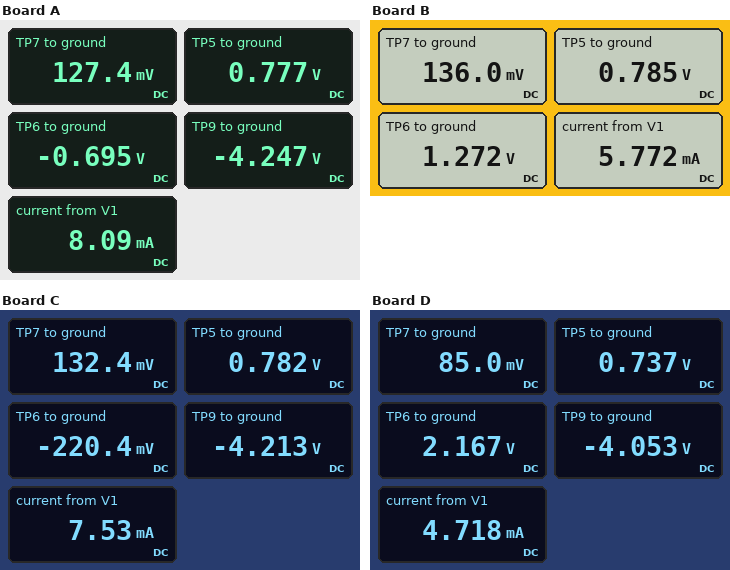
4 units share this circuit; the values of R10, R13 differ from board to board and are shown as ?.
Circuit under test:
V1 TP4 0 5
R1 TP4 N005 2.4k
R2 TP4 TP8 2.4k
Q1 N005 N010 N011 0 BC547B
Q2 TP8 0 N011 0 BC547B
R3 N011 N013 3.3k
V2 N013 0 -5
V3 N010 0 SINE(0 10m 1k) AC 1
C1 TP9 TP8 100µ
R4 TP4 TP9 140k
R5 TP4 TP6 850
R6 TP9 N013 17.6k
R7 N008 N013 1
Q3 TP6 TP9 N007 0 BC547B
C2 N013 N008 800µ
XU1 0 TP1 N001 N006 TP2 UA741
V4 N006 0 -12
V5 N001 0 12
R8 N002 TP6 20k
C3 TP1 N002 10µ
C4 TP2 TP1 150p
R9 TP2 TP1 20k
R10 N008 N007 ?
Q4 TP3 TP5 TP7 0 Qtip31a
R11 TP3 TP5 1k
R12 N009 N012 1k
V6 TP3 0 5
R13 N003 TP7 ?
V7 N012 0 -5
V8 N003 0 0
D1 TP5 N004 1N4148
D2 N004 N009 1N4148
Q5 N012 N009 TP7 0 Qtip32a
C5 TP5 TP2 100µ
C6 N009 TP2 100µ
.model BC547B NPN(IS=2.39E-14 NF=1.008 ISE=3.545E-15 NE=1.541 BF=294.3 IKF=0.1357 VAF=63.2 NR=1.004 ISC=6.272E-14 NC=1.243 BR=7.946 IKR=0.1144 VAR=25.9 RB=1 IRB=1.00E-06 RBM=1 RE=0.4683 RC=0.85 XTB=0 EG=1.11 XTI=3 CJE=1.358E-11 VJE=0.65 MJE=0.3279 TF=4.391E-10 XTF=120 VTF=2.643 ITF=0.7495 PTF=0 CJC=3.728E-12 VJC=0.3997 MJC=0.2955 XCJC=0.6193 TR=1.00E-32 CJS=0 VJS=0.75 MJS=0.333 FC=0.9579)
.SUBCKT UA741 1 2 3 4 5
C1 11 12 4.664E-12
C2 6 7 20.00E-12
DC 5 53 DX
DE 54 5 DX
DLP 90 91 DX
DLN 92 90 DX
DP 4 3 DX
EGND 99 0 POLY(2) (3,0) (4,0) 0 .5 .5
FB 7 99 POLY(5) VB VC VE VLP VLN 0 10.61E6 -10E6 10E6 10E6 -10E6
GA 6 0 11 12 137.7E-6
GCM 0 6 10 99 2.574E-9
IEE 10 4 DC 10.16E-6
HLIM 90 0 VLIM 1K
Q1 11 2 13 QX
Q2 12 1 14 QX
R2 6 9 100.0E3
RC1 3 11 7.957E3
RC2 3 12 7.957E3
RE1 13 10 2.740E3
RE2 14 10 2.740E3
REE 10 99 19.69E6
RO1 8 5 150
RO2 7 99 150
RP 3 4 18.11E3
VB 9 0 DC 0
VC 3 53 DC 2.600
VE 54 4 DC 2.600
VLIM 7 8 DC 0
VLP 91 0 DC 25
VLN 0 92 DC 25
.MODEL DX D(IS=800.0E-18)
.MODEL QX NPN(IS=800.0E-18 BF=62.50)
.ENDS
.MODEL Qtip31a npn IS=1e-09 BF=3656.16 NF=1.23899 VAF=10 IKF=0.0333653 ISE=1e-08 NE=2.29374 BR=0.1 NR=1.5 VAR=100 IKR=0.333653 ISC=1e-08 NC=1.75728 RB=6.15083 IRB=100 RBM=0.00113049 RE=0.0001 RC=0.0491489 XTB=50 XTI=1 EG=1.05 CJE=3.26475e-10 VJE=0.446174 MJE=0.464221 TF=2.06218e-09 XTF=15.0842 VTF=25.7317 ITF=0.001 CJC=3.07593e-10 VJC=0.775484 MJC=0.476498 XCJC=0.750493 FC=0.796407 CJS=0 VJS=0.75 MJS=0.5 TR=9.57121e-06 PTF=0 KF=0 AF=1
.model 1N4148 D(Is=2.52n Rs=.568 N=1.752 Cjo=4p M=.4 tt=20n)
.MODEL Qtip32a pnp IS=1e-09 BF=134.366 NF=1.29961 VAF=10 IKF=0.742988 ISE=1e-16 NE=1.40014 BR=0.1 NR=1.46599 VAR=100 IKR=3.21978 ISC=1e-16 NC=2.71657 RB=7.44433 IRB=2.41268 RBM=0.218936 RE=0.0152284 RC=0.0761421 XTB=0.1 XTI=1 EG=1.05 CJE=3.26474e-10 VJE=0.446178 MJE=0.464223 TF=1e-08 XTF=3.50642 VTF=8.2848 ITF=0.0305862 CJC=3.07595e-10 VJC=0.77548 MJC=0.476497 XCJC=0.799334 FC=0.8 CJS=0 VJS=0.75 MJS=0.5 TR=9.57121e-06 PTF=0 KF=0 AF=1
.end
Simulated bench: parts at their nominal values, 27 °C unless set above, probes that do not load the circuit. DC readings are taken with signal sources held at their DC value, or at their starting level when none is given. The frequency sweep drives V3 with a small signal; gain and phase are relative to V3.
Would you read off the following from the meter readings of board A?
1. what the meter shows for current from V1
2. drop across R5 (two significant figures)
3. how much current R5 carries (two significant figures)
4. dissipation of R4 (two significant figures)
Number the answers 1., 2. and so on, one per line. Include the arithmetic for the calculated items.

1. 8.09 mA
2. 5 V - (-695 mV) = 5.7 V
3. (5 V - (-695 mV)) / 850 Ω = 6.7 mA
4. (5 V - (-4.247 V))^2 / 140 kΩ = 610 µW
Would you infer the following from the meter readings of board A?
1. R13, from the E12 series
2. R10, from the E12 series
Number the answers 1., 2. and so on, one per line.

1. 12 Ω
2. 8.2 Ω
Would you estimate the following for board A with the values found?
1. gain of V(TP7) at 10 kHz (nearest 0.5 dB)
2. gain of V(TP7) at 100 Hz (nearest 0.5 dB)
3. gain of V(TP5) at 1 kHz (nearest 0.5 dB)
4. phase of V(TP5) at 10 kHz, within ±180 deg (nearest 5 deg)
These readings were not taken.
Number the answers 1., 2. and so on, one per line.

1. 59.5 dB
2. 59.0 dB
3. 59.5 dB
4. -15 deg
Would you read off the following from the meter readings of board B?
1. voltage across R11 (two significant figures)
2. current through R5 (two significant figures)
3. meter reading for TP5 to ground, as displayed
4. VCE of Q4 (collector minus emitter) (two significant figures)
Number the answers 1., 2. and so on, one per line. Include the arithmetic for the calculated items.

1. 5 V - 785 mV = 4.2 V
2. (5 V - 1.272 V) / 850 Ω = 4.4 mA
3. 0.785 V
4. 5 V - 136 mV = 4.9 V
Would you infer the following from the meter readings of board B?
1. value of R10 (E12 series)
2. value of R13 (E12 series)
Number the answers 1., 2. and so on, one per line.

1. 47 Ω
2. 18 Ω
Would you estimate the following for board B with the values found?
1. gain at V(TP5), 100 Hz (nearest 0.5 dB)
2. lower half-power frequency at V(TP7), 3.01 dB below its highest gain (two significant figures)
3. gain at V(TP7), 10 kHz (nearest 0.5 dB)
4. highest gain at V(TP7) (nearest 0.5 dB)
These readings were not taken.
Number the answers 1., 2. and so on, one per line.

1. 50.5 dB
2. 2.3 Hz
3. 50.0 dB
4. 50.5 dB
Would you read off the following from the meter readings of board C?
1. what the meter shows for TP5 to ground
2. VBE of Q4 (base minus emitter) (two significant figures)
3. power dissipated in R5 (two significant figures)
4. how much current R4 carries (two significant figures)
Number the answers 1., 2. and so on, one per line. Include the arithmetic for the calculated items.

1. 0.782 V
2. 782 mV - 132.4 mV = 650 mV
3. (5 V - (-220.4 mV))^2 / 850 Ω = 32 mW
4. (5 V - (-4.213 V)) / 140 kΩ = 66 µA
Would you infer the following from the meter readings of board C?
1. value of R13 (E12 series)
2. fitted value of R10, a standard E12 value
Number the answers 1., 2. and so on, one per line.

1. 15 Ω
2. 15 Ω
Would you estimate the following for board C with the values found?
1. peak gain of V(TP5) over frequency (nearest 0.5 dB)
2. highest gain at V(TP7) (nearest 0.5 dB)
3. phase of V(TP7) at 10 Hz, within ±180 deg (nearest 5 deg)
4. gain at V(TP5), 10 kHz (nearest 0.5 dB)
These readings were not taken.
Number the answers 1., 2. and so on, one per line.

1. 57.0 dB
2. 57.0 dB
3. 15 deg
4. 57.0 dB
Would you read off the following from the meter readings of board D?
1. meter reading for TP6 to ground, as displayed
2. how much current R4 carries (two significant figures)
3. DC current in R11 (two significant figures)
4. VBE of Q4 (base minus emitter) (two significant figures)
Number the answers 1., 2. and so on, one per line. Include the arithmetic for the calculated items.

1. 2.167 V
2. (5 V - (-4.053 V)) / 140 kΩ = 65 µA
3. (5 V - 737 mV) / 1 kΩ = 4.3 mA
4. 737 mV - 85 mV = 650 mV
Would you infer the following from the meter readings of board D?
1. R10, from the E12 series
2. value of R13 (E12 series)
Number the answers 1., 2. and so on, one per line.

1. 82 Ω
2. 3.3 Ω
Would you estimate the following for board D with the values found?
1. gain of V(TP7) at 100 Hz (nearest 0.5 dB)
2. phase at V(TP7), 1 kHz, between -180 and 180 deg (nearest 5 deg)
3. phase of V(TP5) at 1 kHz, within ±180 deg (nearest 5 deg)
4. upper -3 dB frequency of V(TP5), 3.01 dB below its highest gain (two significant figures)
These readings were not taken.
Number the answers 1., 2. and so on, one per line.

1. 46.0 dB
2. 0 deg
3. 0 deg
4. 52 kHz
